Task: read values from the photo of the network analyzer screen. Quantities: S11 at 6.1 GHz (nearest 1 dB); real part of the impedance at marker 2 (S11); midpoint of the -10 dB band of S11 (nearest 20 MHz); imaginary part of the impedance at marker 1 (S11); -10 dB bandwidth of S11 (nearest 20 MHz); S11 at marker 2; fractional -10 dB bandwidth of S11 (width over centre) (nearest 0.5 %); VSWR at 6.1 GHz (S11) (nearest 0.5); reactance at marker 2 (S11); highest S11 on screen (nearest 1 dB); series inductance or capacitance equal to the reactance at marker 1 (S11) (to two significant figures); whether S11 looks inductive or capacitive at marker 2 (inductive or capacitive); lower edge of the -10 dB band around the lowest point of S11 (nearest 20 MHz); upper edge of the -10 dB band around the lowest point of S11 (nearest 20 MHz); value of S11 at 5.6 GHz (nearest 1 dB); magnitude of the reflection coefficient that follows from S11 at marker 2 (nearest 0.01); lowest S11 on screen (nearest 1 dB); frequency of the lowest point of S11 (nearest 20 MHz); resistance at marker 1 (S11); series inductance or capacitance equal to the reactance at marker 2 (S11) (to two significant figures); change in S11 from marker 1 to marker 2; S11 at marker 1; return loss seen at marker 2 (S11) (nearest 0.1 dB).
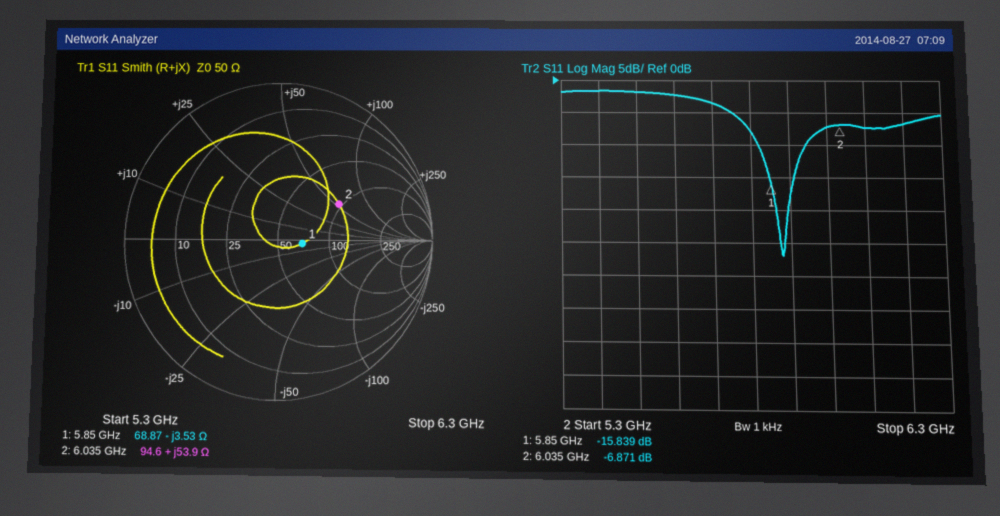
-7 dB
94.6 Ω
5.88 GHz
-3.53 Ω
120 MHz
-6.871 dB
2.0 %
2.5
+53.9 Ω
-2 dB
7.7 pF
inductive
5.82 GHz
5.94 GHz
-2 dB
0.45
-27 dB
5.88 GHz
68.87 Ω
1.4 nH
8.968 dB
-15.839 dB
6.9 dB
